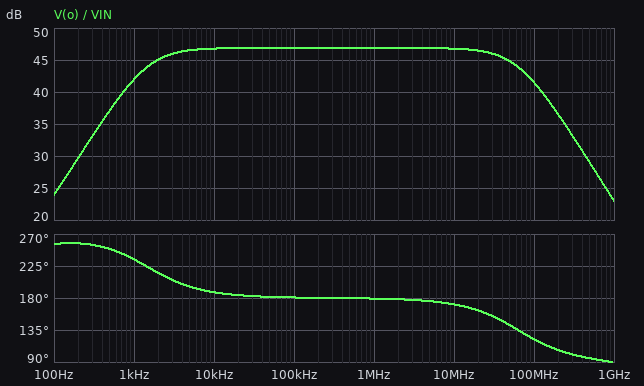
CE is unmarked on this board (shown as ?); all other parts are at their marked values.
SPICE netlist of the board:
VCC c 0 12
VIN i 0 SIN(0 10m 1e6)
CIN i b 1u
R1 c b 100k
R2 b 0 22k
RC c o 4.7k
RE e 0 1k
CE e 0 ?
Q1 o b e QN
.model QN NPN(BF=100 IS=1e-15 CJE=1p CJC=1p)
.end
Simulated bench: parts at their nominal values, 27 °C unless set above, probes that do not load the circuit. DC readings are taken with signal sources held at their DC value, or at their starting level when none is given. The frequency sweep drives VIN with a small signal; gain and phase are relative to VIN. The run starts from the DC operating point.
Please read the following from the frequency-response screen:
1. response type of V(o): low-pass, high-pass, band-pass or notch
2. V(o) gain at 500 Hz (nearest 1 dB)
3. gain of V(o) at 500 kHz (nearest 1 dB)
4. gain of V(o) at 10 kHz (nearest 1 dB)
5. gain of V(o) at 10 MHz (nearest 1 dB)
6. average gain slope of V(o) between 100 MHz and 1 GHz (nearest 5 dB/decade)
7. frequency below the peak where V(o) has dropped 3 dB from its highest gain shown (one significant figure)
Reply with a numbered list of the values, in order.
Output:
1. band-pass
2. 37 dB
3. 47 dB
4. 47 dB
5. 47 dB
6. -20 dB/decade
7. 1 kHz
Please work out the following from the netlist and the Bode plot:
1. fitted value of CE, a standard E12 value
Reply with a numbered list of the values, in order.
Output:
1. 5.6 µF
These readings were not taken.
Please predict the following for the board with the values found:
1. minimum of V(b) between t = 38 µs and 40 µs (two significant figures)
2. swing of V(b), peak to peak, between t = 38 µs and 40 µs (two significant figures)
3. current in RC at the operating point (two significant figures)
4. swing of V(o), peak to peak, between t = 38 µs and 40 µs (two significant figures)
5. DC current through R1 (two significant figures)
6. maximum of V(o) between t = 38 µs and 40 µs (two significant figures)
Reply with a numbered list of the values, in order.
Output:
1. 1.9 V
2. 20 mV
3. 1.2 mA
4. 4.5 V
5. 100 µA
6. 8.2 V
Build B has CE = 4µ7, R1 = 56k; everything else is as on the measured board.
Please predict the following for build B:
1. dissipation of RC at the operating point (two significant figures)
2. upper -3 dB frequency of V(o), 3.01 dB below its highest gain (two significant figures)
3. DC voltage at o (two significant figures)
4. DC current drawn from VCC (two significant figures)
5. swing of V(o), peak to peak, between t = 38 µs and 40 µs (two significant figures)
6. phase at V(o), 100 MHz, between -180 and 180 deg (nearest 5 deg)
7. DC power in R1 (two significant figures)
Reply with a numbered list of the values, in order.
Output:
1. 20 mW
2. 130 MHz
3. 2.2 V
4. 2.2 mA
5. 3.8 V
6. 140 deg
7. 1.5 mW
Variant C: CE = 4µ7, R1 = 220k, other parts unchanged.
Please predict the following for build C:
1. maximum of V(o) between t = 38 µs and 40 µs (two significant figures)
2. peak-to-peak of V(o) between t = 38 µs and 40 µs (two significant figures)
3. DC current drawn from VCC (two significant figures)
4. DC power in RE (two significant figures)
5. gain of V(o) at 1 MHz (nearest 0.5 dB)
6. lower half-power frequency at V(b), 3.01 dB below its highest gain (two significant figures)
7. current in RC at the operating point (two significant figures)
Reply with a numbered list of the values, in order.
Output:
1. 11 V
2. 1.2 V
3. 380 µA
4. 110 µW
5. 35.5 dB
6. 9.8 Hz
7. 330 µA
